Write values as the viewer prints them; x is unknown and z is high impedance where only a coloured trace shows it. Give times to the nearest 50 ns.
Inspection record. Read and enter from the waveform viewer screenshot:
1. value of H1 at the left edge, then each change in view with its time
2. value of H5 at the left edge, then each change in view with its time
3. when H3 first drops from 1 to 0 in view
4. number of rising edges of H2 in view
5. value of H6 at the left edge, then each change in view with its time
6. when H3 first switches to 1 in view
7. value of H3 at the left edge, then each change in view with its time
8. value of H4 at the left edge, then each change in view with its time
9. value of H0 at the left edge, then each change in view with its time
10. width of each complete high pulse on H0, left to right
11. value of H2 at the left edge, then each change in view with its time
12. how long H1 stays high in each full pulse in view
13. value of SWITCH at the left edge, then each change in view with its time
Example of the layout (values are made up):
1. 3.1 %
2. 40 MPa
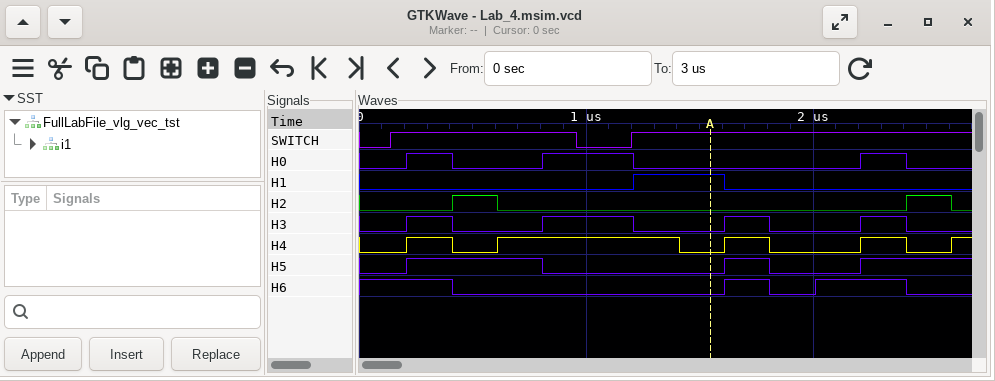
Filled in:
1. 0, 1 at 1200 ns, 0 at 1600 ns
2. 0, 1 at 200 ns, 0 at 800 ns, 1 at 1600 ns, 0 at 1800 ns, 1 at 2200 ns
3. 400 ns
4. 2
5. 1, 0 at 400 ns, 1 at 1600 ns, 0 at 1800 ns, 1 at 2000 ns, 0 at 2400 ns
6. 200 ns
7. 0, 1 at 200 ns, 0 at 400 ns, 1 at 800 ns, 0 at 1200 ns, 1 at 1600 ns, 0 at 1800 ns, 1 at 2200 ns, 0 at 2400 ns
8. 0, 1 at 200 ns, 0 at 400 ns, 1 at 600 ns, 0 at 1400 ns, 1 at 1600 ns, 0 at 1800 ns, 1 at 2200 ns, 0 at 2400 ns, 1 at 2600 ns
9. 0, 1 at 200 ns, 0 at 400 ns, 1 at 800 ns, 0 at 1200 ns, 1 at 2200 ns, 0 at 2400 ns
10. 200 ns, 400 ns, 200 ns
11. 0, 1 at 400 ns, 0 at 600 ns, 1 at 2400 ns, 0 at 2600 ns
12. 400 ns
13. 0, 1 at 150 ns, 0 at 950 ns, 1 at 1200 ns
